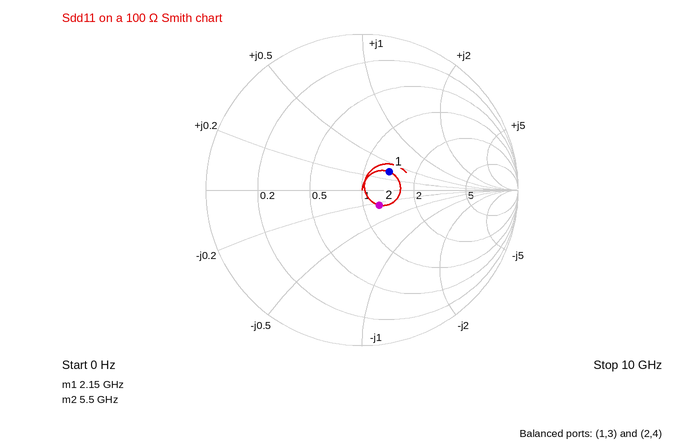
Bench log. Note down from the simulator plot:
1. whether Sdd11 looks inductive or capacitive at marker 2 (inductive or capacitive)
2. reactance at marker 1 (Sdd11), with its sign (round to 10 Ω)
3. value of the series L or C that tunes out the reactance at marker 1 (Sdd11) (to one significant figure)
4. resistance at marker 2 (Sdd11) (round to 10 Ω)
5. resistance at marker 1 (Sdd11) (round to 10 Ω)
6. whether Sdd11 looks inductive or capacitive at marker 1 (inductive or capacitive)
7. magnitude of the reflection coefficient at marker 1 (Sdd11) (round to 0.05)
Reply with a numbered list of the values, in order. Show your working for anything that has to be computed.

1. capacitive
2. +30 Ω
3. C = 1/(2π × 2.15 GHz × 30 Ω) ≈ 2 pF
4. 120 Ω
5. 140 Ω
6. inductive
7. 0.20
